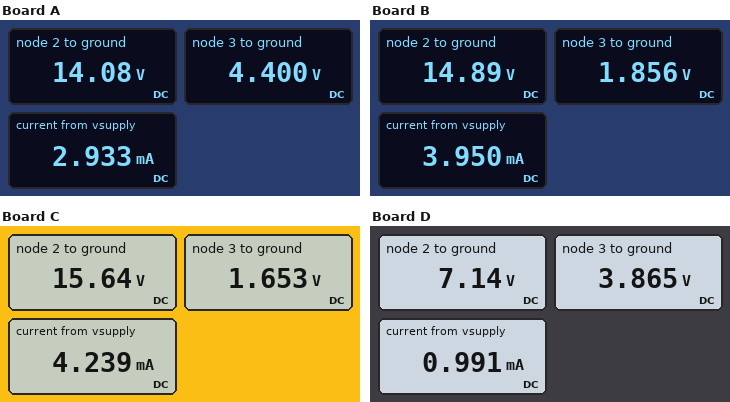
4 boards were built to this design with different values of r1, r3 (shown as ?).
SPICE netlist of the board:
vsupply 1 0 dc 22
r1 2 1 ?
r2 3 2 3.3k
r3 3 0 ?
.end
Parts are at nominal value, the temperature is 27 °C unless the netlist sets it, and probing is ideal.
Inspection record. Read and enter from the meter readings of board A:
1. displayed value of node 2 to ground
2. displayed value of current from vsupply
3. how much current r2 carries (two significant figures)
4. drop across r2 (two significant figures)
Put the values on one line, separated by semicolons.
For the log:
14.08 V; 2.933 mA; 2.9 mA; 9.7 V
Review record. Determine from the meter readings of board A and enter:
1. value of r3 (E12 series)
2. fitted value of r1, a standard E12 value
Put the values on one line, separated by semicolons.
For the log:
1.5 kΩ; 2.7 kΩ
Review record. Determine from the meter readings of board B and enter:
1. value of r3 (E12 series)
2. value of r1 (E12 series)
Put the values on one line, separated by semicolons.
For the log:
470 Ω; 1.8 kΩ
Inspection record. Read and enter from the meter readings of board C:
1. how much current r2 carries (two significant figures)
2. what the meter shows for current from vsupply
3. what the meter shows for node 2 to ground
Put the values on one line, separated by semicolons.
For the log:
4.2 mA; 4.239 mA; 15.64 V
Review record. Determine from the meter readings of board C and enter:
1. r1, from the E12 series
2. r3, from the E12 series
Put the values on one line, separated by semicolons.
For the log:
1.5 kΩ; 390 Ω
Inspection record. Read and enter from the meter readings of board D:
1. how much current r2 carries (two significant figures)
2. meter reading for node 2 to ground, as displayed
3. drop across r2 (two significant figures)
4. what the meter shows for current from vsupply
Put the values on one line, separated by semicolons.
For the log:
990 µA; 7.14 V; 3.3 V; 0.991 mA
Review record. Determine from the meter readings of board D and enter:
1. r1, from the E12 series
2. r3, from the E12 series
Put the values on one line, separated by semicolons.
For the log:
15 kΩ; 3.9 kΩ
